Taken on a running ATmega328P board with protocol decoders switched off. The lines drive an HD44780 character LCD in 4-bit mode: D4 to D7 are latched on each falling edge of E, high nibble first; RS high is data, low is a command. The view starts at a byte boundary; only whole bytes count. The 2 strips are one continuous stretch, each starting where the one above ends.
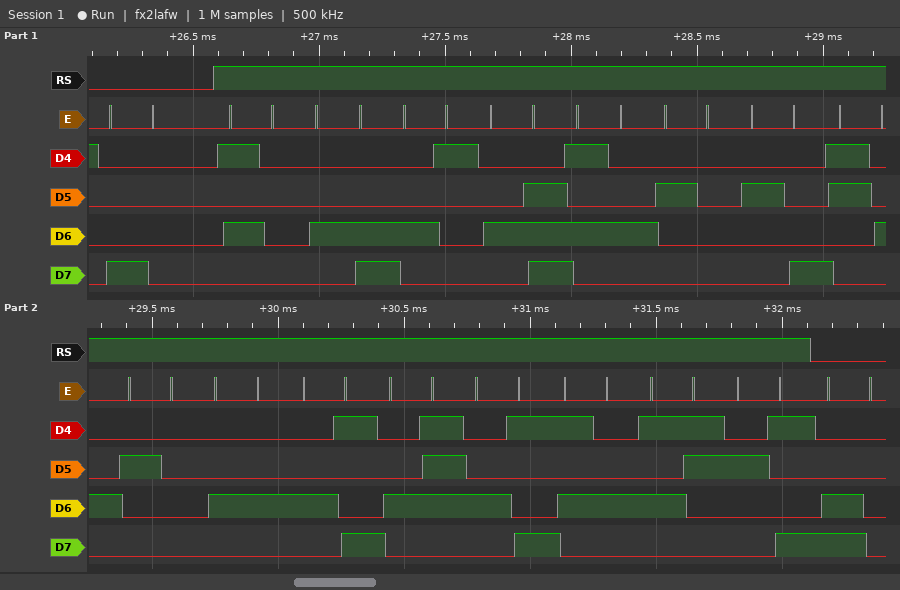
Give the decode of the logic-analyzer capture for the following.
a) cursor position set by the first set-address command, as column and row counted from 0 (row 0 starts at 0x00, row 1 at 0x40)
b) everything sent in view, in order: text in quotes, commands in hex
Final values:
column 0, row 0
0x80 "PLANT (4 DIGITS)" 0xC0
